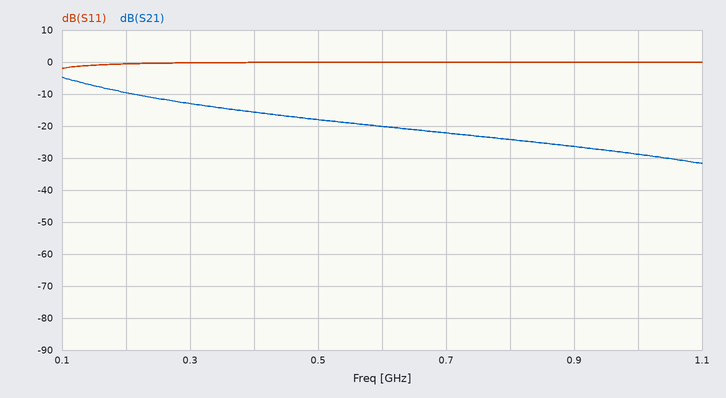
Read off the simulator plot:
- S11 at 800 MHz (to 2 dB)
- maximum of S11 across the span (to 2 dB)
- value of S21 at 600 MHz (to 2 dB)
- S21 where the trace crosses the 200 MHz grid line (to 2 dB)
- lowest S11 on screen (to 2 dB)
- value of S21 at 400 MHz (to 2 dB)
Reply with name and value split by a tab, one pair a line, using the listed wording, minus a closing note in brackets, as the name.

S11 at 800 MHz	0 dB
maximum of S11 across the span	0 dB
value of S21 at 600 MHz	-20 dB
S21 where the trace crosses the 200 MHz grid line	-10 dB
lowest S11 on screen	-2 dB
value of S21 at 400 MHz	-16 dB
